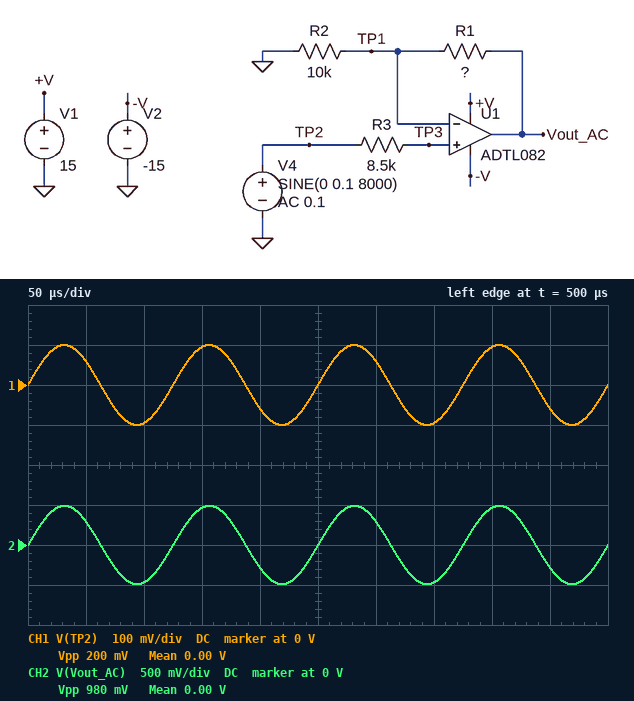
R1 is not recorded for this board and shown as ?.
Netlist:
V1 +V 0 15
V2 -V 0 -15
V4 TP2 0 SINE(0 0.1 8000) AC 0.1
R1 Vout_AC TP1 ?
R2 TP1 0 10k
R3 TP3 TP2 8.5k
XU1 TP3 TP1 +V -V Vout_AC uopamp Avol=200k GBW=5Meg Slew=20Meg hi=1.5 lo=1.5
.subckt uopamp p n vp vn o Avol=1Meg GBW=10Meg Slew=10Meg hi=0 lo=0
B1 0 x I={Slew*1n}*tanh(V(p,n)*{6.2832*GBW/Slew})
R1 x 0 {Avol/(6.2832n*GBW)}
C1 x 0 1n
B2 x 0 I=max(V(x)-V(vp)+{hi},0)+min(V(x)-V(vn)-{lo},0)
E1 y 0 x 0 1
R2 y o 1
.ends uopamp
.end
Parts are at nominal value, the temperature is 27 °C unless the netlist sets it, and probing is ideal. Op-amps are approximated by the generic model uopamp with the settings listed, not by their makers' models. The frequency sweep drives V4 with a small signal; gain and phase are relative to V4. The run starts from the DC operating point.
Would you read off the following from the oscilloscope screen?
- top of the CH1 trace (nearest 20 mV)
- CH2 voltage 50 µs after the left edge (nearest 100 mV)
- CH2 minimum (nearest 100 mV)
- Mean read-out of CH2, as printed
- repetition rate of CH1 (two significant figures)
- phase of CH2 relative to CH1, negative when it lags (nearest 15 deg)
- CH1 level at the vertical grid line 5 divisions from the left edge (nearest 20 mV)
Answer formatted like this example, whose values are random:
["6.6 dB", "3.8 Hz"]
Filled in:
["100 mV", "300 mV", "-500 mV", "0.00 V", "8.0 kHz", "0 deg", "0 V"]
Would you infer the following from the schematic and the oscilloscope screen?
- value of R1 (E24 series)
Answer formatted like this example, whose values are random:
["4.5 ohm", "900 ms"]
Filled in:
["39 kΩ"]
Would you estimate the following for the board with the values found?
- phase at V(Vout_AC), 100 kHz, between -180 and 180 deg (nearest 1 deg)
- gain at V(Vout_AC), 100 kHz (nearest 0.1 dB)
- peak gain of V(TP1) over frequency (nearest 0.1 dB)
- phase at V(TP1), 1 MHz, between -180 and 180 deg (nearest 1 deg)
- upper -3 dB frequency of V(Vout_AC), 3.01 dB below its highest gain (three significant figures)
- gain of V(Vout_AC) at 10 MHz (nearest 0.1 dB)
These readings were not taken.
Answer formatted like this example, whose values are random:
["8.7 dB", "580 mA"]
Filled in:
["-6 deg", "13.8 dB", "0 dB", "-44 deg", "1.02 MHz", "-6.1 dB"]
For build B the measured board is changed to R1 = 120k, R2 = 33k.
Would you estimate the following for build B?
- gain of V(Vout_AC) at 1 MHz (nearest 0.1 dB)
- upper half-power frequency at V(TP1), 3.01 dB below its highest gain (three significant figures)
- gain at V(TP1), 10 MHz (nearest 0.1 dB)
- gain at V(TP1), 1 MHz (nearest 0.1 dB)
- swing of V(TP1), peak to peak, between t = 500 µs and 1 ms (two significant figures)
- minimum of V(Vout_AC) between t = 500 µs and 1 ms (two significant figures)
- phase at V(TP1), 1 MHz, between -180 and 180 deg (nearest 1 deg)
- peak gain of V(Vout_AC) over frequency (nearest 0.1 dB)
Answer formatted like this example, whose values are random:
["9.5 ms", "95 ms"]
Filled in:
["10.6 dB", "1.08 MHz", "-19.4 dB", "-2.7 dB", "200 mV", "-460 mV", "-43 deg", "13.3 dB"]
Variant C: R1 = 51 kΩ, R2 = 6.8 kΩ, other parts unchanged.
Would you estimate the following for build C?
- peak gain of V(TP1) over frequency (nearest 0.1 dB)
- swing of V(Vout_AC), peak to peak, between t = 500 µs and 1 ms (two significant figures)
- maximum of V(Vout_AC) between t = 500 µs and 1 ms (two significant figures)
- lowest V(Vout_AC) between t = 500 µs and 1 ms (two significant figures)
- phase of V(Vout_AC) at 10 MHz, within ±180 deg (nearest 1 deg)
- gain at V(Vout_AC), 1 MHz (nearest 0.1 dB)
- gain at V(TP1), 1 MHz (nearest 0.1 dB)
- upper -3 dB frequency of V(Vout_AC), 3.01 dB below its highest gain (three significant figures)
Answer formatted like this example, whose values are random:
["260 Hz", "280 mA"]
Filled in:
["0 dB", "1.7 V", "850 mV", "-850 mV", "-87 deg", "12.7 dB", "-5.9 dB", "588 kHz"]
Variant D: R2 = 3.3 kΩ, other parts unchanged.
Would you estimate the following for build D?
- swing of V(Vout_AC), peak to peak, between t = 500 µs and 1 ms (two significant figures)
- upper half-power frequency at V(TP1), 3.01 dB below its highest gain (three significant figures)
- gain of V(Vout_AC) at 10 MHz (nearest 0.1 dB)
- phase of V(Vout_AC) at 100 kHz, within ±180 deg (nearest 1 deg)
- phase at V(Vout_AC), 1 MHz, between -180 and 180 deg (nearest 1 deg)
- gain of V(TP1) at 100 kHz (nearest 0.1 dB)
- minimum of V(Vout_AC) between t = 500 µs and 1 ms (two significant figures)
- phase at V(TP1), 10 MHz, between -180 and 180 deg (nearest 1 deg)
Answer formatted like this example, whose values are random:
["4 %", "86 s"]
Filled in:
["2.6 V", "390 kHz", "-6.0 dB", "-14 deg", "-69 deg", "-0.3 dB", "-1.3 V", "-88 deg"]
